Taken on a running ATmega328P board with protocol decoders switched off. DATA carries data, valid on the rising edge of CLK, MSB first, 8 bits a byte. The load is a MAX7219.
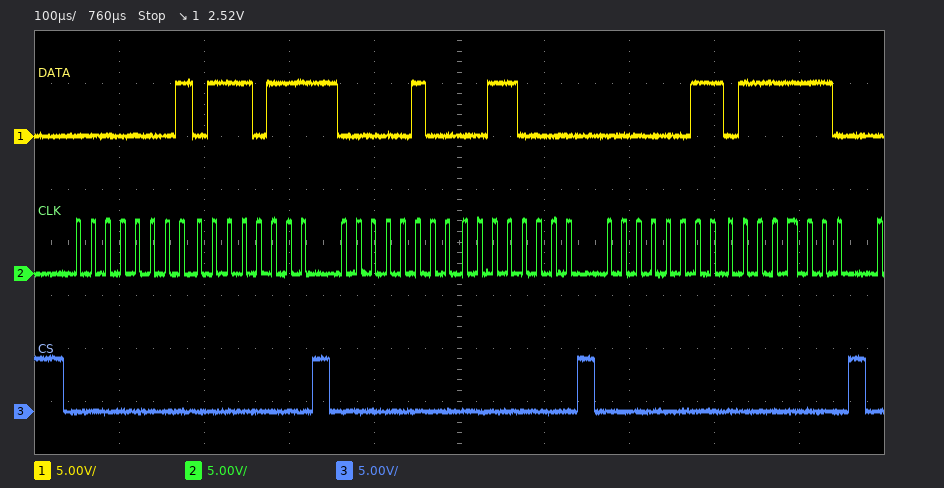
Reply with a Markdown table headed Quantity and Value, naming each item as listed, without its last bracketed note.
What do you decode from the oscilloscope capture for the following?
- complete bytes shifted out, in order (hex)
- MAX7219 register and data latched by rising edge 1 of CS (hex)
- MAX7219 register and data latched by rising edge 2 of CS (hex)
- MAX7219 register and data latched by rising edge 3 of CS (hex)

| Quantity | Value |
|---|---|
| complete bytes shifted out, in order | 01 77 04 30 03 7E |
| MAX7219 register and data latched by rising edge 1 of CS | register 0x1, data 0x77 |
| MAX7219 register and data latched by rising edge 2 of CS | register 0x4, data 0x30 |
| MAX7219 register and data latched by rising edge 3 of CS | register 0x3, data 0x7E |
